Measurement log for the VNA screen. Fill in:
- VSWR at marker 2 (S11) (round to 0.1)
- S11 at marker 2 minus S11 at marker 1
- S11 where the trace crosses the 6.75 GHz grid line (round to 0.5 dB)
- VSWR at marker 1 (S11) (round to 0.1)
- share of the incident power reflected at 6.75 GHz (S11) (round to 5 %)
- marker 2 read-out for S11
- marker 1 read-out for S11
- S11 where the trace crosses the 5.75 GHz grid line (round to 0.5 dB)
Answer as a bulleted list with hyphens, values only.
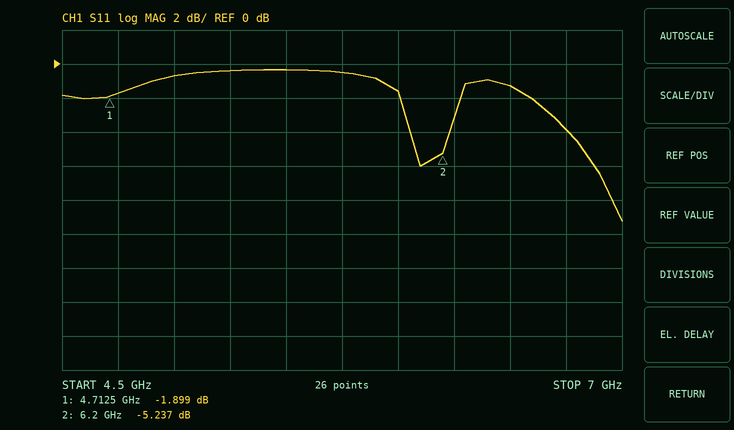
- 3.4
- -3.338 dB
- -4.0 dB
- 9.2
- 40 %
- -5.237 dB
- -1.899 dB
- -0.5 dB
